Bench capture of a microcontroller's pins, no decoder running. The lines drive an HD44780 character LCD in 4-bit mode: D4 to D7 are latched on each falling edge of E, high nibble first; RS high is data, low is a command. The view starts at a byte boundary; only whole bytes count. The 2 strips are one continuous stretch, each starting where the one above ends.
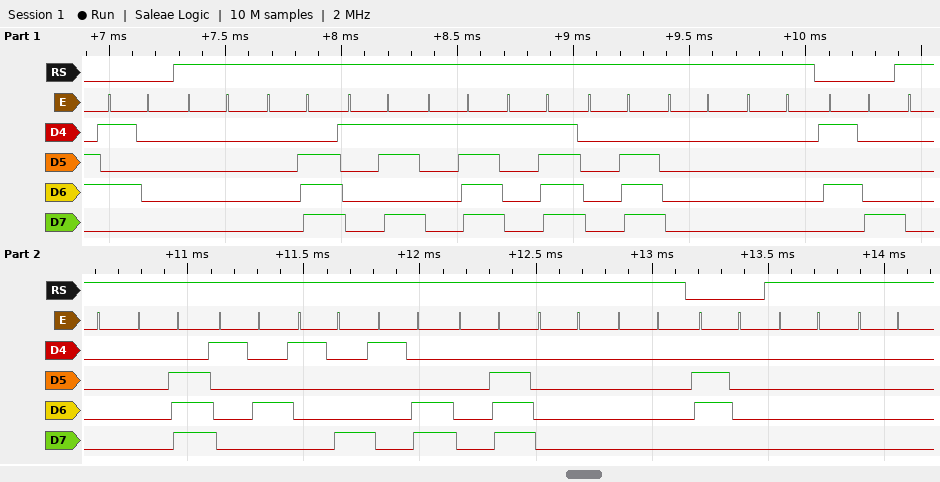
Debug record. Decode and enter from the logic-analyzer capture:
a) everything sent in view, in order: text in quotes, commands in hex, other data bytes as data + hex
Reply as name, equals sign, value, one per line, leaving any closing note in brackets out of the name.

everything sent in view, in order: text in quotes, commands in hex, other data bytes as data + hex = 0x50 data 00 0E 1B 1F 1F 0E 00 00 0x58 data 00 0E 14 18 1C 0E 00 00 0x60 data 00 00
